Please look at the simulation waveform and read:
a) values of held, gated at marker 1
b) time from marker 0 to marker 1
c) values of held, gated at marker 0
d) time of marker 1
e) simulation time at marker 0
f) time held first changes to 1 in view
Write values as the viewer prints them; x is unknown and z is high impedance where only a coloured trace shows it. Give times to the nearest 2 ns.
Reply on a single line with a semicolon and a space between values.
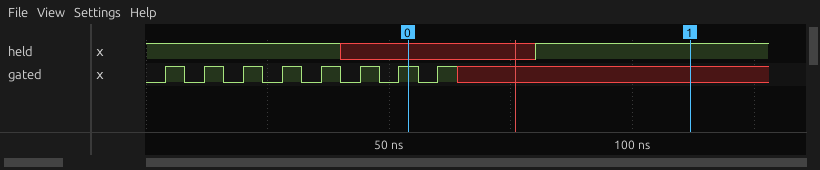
held=1, gated=x; 58 ns; held=x, gated=1; 112 ns; 54 ns; 80 ns
